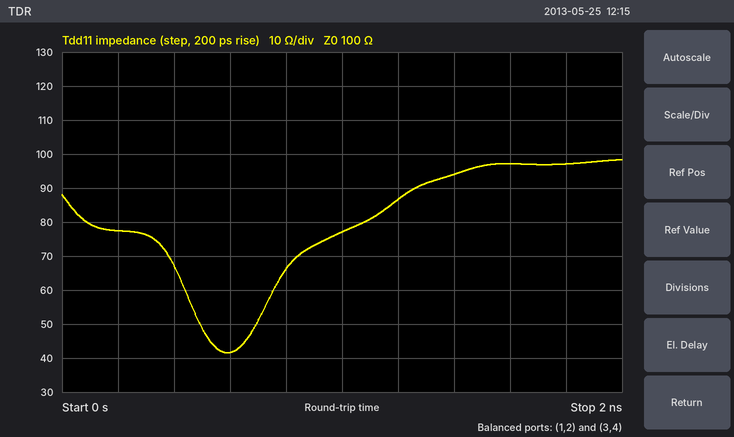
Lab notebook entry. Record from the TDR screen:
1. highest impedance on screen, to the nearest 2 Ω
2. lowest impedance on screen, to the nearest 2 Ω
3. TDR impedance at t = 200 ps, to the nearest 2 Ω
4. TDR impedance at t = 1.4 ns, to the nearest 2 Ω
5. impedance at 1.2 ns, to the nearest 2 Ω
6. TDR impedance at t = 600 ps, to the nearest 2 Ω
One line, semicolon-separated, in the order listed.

98 Ω; 42 Ω; 78 Ω; 94 Ω; 86 Ω; 42 Ω
